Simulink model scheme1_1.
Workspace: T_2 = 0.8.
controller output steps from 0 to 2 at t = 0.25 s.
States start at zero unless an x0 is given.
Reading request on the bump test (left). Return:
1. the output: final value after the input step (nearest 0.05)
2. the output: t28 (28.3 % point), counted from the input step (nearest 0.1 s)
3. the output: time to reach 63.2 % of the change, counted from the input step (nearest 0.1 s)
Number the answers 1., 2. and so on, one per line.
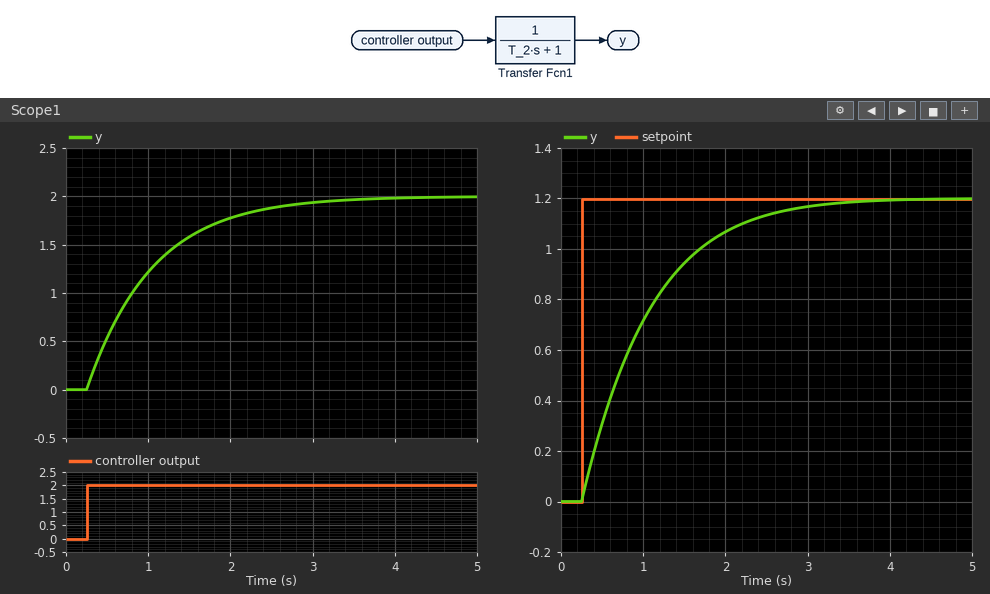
1. 2.00
2. 0.3 s
3. 0.8 s
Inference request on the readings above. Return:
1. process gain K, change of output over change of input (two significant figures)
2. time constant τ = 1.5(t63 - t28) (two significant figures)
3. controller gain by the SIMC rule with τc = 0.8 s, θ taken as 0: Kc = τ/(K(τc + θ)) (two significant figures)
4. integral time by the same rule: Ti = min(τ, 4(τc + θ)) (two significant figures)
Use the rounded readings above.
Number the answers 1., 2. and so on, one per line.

1. 1.0
2. 0.75 s
3. 0.94
4. 0.75 s
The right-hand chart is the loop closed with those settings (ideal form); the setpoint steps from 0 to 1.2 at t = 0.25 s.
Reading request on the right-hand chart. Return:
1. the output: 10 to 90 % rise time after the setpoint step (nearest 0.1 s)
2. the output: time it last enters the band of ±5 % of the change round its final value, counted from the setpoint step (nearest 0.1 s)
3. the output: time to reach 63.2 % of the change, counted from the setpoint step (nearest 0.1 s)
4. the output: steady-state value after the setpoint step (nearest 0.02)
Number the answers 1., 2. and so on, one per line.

1. 1.7 s
2. 2.3 s
3. 0.8 s
4. 1.20
